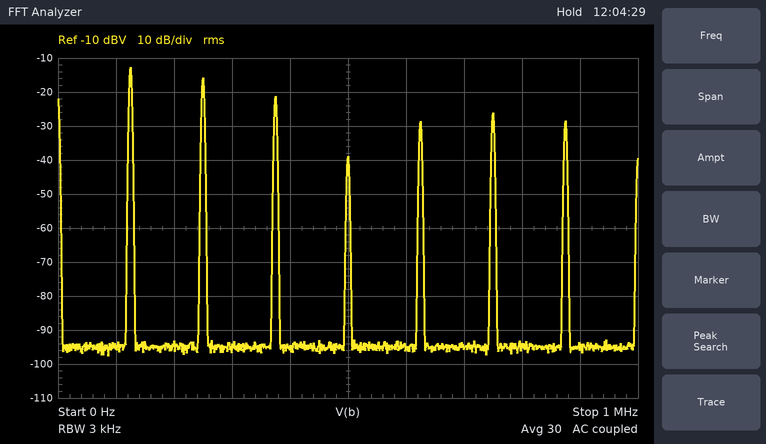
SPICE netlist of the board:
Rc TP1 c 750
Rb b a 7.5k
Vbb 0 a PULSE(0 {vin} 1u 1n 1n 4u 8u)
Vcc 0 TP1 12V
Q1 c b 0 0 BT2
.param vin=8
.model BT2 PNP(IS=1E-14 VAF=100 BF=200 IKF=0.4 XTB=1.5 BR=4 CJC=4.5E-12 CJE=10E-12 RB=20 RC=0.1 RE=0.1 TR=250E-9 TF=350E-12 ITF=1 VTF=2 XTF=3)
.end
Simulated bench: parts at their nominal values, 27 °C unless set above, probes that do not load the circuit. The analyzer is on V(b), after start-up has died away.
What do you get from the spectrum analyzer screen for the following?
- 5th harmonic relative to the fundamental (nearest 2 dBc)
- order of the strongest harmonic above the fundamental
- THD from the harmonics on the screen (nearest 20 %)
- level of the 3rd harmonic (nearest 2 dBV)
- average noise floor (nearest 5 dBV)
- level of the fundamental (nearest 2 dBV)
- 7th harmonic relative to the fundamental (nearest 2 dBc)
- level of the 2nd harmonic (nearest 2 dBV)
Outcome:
-16 dBc
2
80 %
-22 dBV
-95 dBV
-12 dBV
-16 dBc
-16 dBV
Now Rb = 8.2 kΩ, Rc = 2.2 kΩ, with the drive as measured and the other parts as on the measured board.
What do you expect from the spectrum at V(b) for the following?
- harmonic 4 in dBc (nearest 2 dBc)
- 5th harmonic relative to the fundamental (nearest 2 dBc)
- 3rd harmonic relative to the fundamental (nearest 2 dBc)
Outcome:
-10 dBc
-20 dBc
-4 dBc
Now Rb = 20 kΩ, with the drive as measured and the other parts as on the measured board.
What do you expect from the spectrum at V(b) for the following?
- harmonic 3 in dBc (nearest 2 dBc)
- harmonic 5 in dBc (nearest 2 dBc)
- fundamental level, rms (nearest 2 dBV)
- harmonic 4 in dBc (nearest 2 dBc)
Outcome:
-12 dBc
-14 dBc
-12 dBV
-24 dBc
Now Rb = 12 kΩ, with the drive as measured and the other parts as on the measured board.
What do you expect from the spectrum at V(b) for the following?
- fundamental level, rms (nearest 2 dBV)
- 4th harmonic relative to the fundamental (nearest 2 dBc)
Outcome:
-12 dBV
-32 dBc
